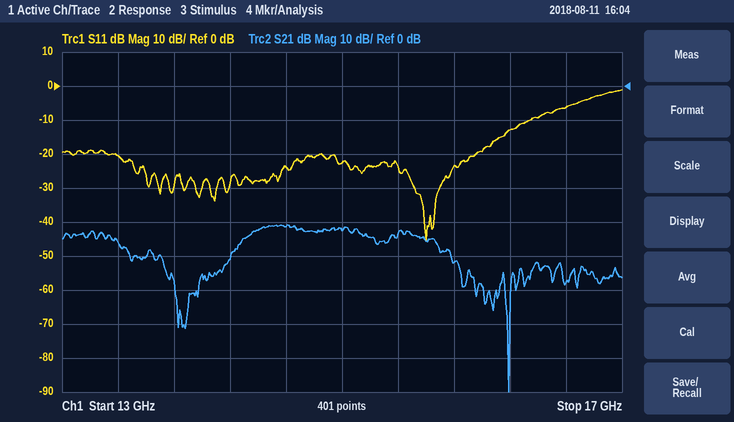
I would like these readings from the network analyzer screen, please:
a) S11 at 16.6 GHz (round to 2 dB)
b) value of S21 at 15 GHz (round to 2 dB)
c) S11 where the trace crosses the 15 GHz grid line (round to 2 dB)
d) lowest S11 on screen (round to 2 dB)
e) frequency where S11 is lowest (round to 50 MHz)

-6 dB
-42 dB
-22 dB
-46 dB
15.60 GHz
